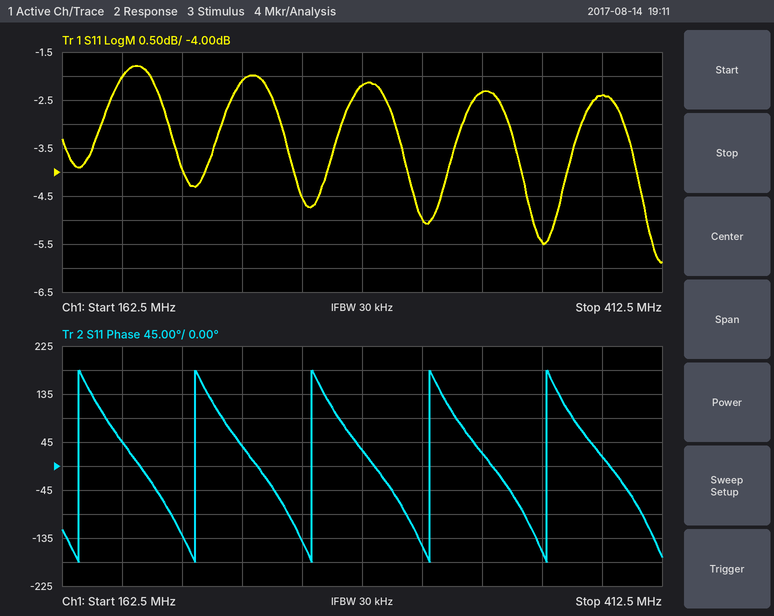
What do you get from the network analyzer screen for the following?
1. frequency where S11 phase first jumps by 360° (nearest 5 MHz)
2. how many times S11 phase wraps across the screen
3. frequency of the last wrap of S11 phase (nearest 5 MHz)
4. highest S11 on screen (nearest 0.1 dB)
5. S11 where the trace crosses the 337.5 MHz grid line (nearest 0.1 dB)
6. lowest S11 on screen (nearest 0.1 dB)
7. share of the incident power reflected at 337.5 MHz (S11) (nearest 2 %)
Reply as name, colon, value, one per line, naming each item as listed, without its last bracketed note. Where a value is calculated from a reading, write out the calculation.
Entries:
frequency where S11 phase first jumps by 360°: 170 MHz
how many times S11 phase wraps across the screen: 5
frequency of the last wrap of S11 phase: 365 MHz
highest S11 on screen: -1.8 dB
S11 where the trace crosses the 337.5 MHz grid line: -2.3 dB
lowest S11 on screen: -5.9 dB
share of the incident power reflected at 337.5 MHz (S11): 10^(-2.3/10) ≈ 58.9 %, so 58 % to the nearest 2 %
